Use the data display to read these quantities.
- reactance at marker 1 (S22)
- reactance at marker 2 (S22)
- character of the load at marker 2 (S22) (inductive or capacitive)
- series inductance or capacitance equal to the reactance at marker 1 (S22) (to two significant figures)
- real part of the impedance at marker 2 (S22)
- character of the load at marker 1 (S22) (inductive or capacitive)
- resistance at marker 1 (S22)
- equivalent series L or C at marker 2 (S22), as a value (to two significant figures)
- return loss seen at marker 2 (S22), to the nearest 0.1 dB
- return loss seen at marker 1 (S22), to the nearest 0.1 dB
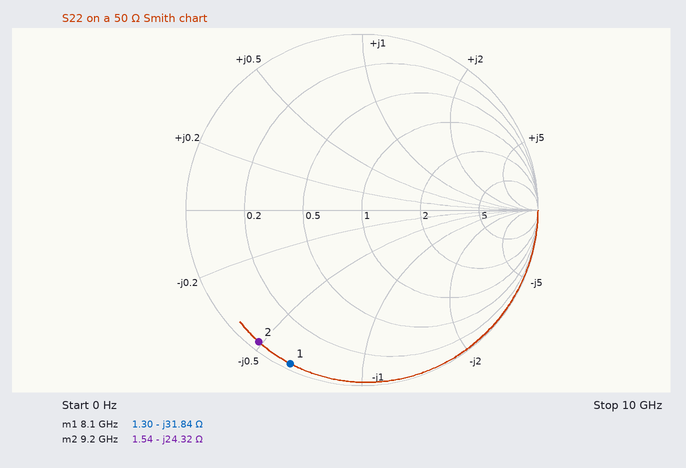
-31.84 Ω
-24.32 Ω
capacitive
620 fF
1.54 Ω
capacitive
1.30 Ω
710 fF
0.4 dB
0.3 dB
